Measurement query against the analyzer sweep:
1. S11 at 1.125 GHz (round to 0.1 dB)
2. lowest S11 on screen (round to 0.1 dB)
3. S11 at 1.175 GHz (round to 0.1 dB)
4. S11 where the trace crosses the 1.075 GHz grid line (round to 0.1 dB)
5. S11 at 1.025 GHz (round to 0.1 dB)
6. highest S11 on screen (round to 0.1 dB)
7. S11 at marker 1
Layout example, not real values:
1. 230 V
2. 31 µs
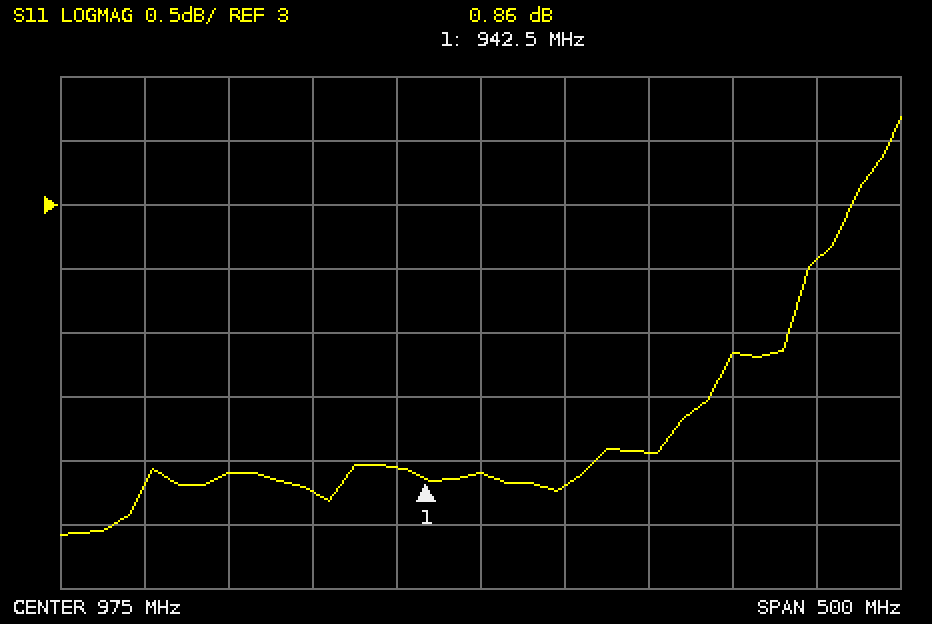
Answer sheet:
1. 1.8 dB
2. 0.4 dB
3. 2.6 dB
4. 1.1 dB
5. 0.8 dB
6. 3.7 dB
7. 0.86 dB
